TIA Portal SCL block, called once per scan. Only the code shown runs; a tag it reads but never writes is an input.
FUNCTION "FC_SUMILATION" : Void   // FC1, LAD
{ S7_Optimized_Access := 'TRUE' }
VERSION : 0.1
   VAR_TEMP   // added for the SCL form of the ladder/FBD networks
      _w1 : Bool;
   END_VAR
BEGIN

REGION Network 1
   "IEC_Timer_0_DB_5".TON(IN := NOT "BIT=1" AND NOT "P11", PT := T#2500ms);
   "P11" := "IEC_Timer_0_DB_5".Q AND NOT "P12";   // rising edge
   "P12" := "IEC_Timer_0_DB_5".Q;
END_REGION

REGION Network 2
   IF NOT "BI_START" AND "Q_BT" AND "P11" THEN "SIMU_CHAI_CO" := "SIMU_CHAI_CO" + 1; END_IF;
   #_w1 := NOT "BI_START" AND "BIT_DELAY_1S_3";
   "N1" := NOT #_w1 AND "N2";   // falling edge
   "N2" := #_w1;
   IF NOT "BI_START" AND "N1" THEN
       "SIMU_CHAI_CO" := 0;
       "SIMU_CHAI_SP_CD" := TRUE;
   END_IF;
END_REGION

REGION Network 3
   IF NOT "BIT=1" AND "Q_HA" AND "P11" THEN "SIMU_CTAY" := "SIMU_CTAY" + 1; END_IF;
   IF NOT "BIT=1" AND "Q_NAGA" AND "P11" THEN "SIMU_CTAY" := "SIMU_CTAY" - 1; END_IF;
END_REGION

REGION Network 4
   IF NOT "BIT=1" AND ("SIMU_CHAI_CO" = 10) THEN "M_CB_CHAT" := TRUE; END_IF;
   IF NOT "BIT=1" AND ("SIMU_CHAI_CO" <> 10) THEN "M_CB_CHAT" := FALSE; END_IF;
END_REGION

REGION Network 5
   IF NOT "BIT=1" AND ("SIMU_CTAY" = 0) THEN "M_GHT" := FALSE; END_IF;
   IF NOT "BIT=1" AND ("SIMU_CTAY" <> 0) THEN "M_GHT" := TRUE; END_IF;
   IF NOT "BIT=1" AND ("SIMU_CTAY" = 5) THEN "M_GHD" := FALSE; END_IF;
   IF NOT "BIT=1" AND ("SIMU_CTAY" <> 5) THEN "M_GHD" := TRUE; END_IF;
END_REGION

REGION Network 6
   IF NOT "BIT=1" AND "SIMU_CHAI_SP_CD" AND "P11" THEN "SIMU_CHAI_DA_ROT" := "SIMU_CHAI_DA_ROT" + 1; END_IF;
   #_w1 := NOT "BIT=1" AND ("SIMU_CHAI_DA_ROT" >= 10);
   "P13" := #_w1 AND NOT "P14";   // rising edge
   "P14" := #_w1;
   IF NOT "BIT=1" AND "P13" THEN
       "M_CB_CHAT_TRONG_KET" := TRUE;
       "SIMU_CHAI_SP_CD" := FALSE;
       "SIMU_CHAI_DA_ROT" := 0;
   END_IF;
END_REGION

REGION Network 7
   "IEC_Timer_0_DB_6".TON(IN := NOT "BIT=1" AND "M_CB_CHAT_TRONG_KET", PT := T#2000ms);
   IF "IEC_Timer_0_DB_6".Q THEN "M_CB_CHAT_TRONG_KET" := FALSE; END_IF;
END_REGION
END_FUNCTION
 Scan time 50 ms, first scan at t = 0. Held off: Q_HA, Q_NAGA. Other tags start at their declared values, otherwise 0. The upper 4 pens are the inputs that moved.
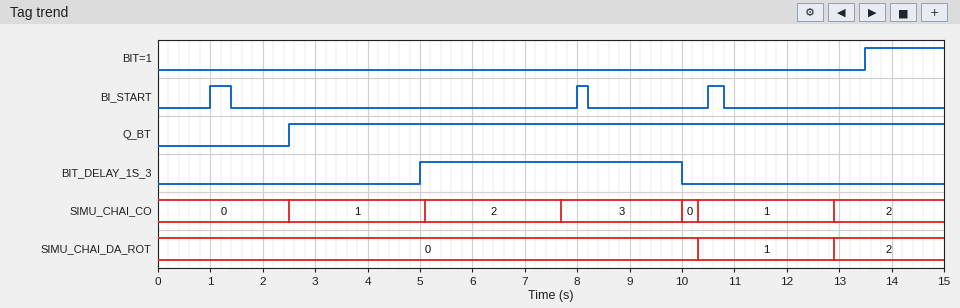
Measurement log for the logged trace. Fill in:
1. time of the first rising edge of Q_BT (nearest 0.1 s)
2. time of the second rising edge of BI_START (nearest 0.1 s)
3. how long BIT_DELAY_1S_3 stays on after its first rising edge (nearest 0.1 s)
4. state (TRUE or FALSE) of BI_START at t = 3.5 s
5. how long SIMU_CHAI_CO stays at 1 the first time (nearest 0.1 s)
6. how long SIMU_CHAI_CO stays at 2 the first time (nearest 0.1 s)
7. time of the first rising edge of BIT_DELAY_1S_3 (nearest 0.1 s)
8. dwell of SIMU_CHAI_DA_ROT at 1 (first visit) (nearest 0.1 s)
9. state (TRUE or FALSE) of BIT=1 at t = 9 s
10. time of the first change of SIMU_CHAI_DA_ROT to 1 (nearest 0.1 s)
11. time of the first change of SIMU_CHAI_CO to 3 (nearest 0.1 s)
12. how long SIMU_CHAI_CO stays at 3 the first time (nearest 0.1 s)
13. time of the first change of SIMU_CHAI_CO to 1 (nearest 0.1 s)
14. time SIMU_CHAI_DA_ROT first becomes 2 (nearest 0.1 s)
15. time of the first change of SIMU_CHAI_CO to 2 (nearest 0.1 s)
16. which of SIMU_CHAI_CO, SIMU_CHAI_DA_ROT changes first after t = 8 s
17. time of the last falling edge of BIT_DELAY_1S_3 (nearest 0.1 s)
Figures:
2.5 s
8.0 s
5.0 s
FALSE
2.6 s
2.6 s
5.0 s
2.6 s
FALSE
10.3 s
7.7 s
2.3 s
2.5 s
12.9 s
5.1 s
SIMU_CHAI_CO
10.0 s
